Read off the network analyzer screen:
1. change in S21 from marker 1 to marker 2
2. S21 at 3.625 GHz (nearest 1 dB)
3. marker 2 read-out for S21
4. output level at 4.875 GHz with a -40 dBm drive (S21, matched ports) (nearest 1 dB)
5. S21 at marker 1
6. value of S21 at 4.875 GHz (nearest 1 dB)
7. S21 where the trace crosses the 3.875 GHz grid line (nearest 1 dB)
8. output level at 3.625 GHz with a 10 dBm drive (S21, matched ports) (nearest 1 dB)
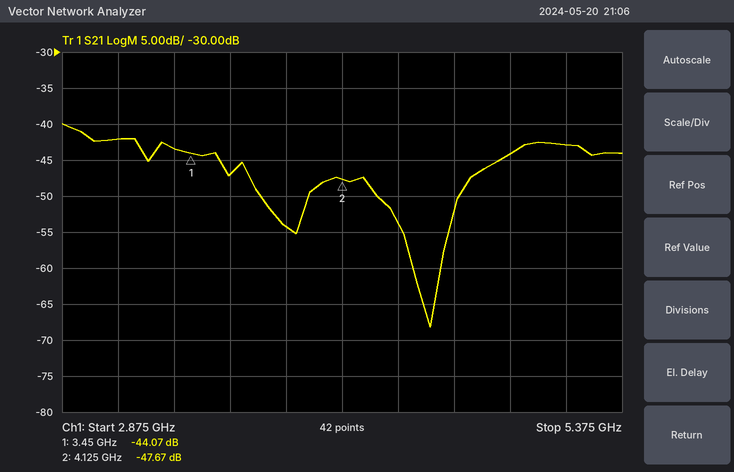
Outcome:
-3.60 dB
-47 dB
-47.67 dB
-84 dBm
-44.07 dB
-44 dB
-54 dB
-37 dBm
